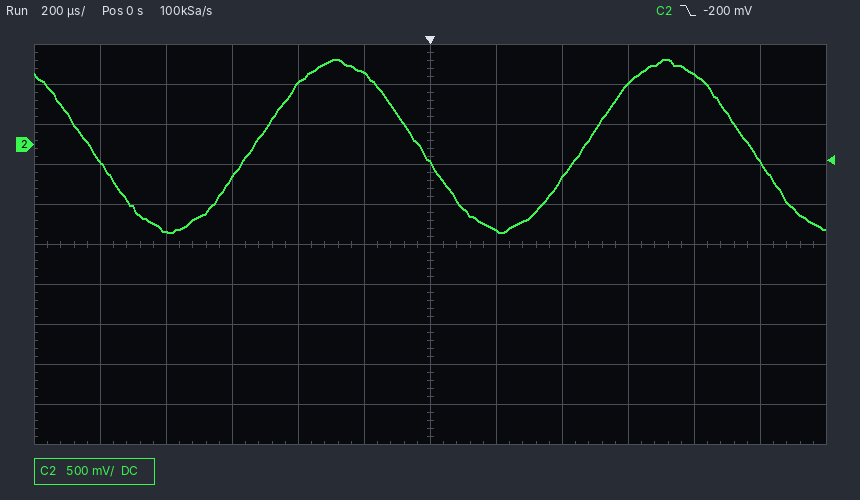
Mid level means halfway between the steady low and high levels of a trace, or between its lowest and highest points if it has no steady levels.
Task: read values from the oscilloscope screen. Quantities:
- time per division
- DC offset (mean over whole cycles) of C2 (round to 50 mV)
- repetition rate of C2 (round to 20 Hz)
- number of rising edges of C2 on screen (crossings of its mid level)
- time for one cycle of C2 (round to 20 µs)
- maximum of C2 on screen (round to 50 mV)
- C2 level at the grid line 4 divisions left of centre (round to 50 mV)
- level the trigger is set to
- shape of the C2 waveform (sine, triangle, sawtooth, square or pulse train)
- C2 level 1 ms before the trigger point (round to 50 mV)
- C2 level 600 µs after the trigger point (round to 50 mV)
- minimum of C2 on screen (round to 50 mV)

200 µs
0 mV
1.00 kHz
2
1.00 ms
1.05 V
-1.10 V
-200 mV
sine
-200 mV
750 mV
-1.10 V
